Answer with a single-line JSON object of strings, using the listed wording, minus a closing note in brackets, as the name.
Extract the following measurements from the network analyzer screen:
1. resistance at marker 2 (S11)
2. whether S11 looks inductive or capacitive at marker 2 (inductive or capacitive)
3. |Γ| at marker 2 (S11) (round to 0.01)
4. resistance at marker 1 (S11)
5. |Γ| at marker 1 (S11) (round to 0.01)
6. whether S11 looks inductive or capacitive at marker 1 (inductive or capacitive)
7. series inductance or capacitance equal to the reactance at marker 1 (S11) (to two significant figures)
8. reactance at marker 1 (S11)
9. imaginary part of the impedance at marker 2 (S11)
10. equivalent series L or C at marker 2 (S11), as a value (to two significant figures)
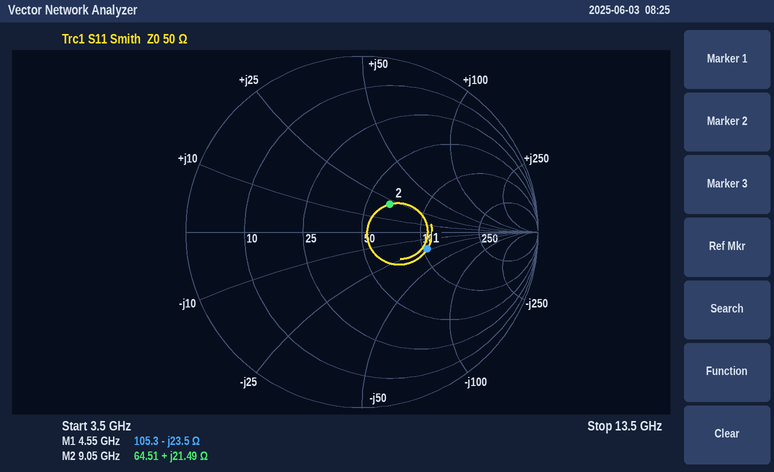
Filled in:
{"resistance at marker 2": "64.51 Ω", "whether S11 looks inductive or capacitive at marker 2": "inductive", "|Γ| at marker 2 (S11)": "0.22", "resistance at marker 1": "105.3 Ω", "|Γ| at marker 1 (S11)": "0.38", "whether S11 looks inductive or capacitive at marker 1": "capacitive", "series inductance or capacitance equal to the reactance at marker 1 (S11)": "1.5 pF", "reactance at marker 1": "-23.5 Ω", "imaginary part of the impedance at marker 2": "+21.49 Ω", "equivalent series L or C at marker 2 (S11), as a value": "380 pH"}
